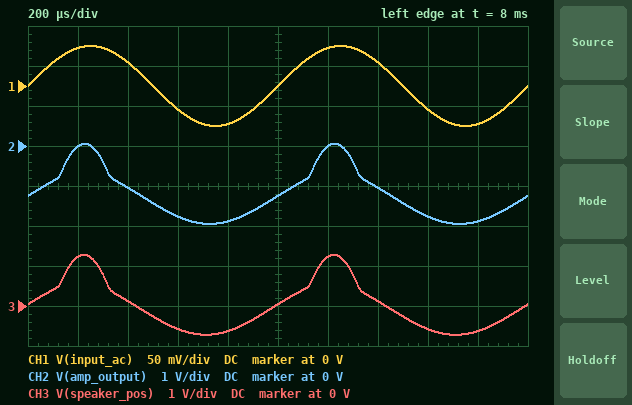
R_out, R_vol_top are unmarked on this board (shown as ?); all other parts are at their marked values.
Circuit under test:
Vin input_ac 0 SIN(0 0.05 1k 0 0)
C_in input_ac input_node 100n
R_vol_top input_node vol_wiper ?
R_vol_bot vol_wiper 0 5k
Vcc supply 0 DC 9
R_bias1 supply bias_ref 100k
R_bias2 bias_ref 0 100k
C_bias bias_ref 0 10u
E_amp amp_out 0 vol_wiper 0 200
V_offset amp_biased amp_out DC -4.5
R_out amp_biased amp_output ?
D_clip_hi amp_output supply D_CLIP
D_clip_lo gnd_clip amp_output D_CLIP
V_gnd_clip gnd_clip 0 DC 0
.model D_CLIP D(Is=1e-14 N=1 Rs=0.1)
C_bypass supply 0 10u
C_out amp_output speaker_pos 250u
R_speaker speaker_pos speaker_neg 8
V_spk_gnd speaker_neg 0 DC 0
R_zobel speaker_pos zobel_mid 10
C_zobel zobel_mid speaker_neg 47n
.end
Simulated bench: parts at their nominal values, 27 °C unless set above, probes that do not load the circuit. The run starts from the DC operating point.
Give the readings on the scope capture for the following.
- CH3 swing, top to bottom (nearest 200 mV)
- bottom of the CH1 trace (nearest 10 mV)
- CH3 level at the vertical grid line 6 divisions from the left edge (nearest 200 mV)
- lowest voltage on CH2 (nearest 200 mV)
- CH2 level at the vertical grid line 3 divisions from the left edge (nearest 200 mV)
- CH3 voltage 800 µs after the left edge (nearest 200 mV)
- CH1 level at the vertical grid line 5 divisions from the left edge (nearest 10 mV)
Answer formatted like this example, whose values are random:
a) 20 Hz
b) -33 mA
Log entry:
a) 2.0 V
b) -50 mV
c) 1.2 V
d) -2.0 V
e) -1.8 V
f) -600 mV
g) 0 V
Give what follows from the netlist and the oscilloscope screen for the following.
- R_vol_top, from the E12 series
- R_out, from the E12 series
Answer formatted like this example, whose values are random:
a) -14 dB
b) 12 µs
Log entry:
a) 5.6 kΩ
b) 0.68 Ω
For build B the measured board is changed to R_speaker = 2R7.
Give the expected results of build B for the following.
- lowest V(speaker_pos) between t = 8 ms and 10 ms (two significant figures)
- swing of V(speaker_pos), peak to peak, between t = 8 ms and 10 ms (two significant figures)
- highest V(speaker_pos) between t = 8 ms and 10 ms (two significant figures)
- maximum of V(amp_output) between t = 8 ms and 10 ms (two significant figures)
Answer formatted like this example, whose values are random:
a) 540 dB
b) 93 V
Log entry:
a) -670 mV
b) 1.8 V
c) 1.1 V
d) -110 mV
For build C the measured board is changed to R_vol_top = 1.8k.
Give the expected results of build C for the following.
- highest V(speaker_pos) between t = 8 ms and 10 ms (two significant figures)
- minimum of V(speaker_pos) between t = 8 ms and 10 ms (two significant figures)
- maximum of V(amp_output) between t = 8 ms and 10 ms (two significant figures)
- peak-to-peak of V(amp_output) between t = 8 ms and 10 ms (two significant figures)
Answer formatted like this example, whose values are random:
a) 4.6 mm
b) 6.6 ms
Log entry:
a) 3.1 V
b) -1.5 V
c) 2.4 V
d) 4.7 V
